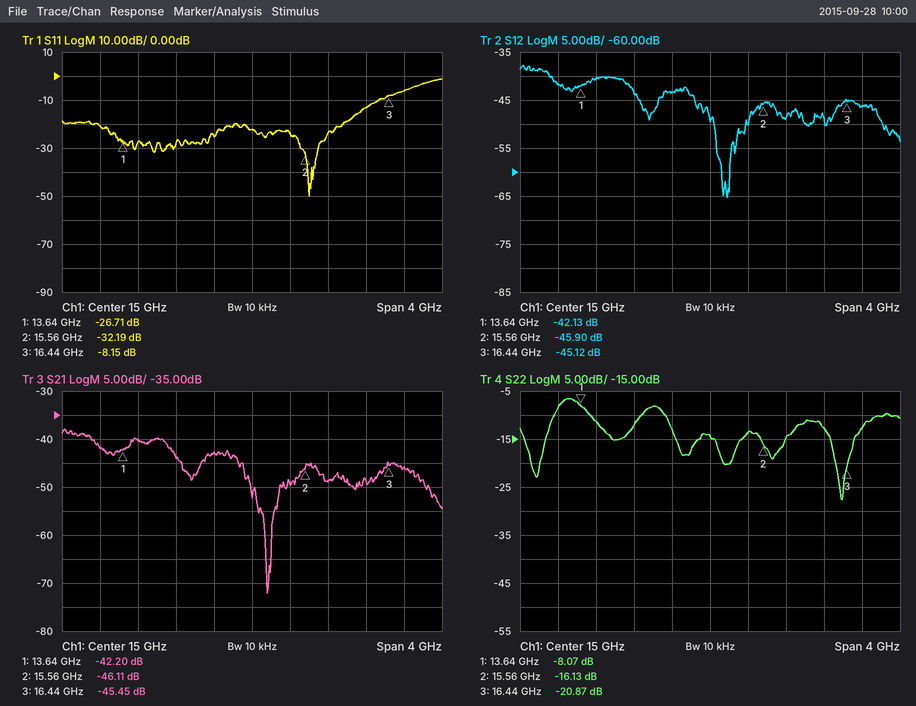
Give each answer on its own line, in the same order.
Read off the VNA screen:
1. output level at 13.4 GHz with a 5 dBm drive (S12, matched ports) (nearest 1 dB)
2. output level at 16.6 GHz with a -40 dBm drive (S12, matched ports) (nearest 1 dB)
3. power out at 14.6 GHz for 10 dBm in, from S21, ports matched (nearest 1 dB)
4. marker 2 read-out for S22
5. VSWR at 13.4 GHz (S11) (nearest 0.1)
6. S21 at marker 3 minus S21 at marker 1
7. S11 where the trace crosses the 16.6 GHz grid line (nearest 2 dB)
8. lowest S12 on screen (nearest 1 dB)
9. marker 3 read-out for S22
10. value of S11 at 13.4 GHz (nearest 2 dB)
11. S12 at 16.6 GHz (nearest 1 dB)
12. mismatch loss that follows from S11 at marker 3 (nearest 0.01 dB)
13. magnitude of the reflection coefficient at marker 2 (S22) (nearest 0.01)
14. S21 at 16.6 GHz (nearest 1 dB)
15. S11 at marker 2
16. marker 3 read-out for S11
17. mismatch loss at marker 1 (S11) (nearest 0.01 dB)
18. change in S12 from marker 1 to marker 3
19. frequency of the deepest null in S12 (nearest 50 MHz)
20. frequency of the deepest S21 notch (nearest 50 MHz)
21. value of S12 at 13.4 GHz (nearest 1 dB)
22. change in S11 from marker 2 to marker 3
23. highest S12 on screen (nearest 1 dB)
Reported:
-37 dBm
-86 dBm
-33 dBm
-16.13 dB
1.2
-3.25 dB
-6 dB
-65 dB
-20.87 dB
-20 dB
-46 dB
0.72 dB
0.16
-46 dB
-32.19 dB
-8.15 dB
0.01 dB
-2.99 dB
15.20 GHz
15.15 GHz
-42 dB
24.04 dB
-38 dB
